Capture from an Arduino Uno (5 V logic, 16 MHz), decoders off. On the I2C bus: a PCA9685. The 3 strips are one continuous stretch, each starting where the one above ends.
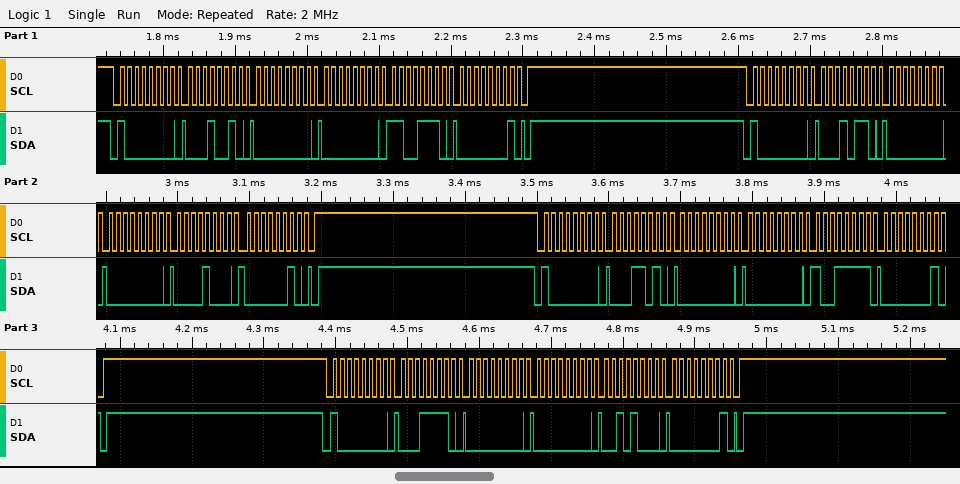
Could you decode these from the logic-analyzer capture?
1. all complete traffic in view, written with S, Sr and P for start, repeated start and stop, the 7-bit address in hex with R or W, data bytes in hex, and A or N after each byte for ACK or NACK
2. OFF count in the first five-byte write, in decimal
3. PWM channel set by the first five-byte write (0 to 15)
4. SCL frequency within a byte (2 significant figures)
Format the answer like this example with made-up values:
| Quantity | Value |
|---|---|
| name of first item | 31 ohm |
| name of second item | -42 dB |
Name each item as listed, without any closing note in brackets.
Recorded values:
| Quantity | Value |
|---|---|
| all complete traffic in view, written with S, Sr and P for start, repeated start and stop, the 7-bit address in hex with R or W, data bytes in hex, and A or N after each byte for ACK or NACK | S 40W A 12 A 00 A 00 A CE A 01 A P S 40W A 16 A 00 A 00 A 08 A 02 A P S 40W A 1A A 00 A 00 A 9F A 01 A P S 40W A 1E A 00 A 00 A 28 A 01 A P |
| OFF count in the first five-byte write, in decimal | 462 |
| PWM channel set by the first five-byte write | 3 |
| SCL frequency within a byte | 100 kHz |
